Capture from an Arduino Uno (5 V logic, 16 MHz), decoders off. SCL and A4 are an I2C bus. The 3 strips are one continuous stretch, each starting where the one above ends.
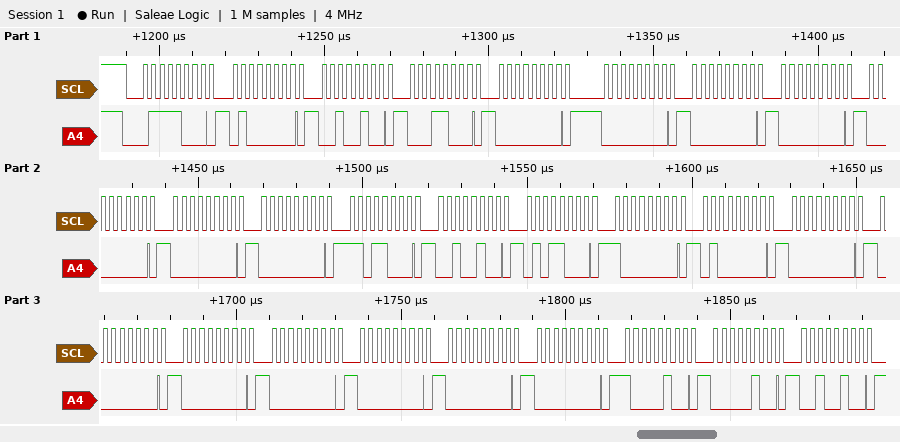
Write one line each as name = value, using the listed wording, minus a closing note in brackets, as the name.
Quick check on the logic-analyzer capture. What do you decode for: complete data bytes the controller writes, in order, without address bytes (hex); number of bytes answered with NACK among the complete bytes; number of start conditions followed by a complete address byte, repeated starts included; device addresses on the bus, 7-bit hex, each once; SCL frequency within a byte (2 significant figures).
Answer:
complete data bytes the controller writes, in order, without address bytes = 40 24 18 00 00 00 00 00 00 00 D8 24 58 80 40 00 00 00 00 00 00 00 84 04 24
number of bytes answered with NACK among the complete bytes = 0
number of start conditions followed by a complete address byte, repeated starts included = 1
device addresses on the bus, 7-bit hex, each once = 0x3C
SCL frequency within a byte = 400 kHz
